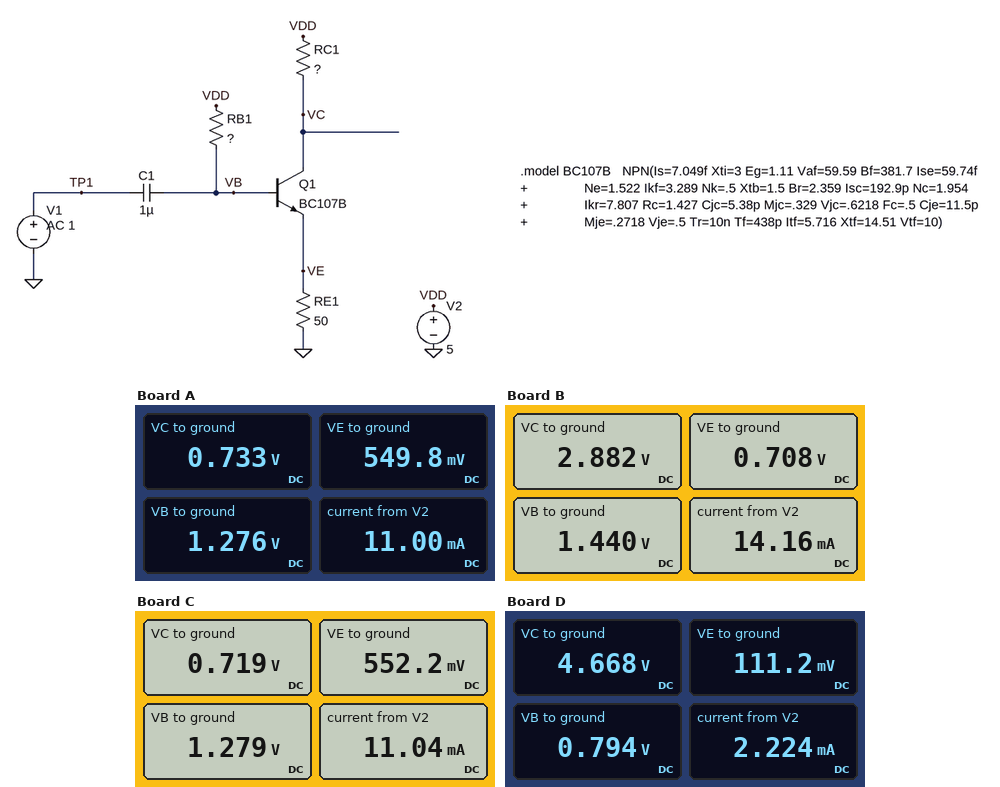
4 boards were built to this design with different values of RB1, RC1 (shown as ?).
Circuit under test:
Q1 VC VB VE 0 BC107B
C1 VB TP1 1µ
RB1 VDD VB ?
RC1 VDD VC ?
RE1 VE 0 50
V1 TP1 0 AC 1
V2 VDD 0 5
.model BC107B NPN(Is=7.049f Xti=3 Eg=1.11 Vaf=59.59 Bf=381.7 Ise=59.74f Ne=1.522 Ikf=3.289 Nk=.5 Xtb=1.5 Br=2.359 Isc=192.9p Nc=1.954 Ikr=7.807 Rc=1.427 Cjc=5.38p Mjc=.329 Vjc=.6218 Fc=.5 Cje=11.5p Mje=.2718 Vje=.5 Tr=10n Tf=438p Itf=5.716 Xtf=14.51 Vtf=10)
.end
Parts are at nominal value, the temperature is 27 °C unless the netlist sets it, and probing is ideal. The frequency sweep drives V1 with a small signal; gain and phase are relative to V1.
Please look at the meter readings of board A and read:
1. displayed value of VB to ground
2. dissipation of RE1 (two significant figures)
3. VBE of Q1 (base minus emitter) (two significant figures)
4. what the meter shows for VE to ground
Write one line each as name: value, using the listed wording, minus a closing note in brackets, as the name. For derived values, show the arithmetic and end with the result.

displayed value of VB to ground: 1.276 V
dissipation of RE1: (549.8 mV)^2 / 50 Ω = 6.0 mW
VBE of Q1 (base minus emitter): 1.276 V - 549.8 mV = 730 mV
what the meter shows for VE to ground: 549.8 mV
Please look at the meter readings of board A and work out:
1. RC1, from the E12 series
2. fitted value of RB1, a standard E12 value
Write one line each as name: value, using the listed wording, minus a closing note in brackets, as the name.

RC1, from the E12 series: 390 Ω
fitted value of RB1, a standard E12 value: 68 kΩ
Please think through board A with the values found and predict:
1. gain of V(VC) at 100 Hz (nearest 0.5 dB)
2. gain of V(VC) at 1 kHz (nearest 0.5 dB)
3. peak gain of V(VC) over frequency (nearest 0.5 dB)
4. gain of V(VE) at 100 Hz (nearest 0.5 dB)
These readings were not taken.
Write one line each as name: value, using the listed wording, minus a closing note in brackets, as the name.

gain of V(VC) at 100 Hz: 0 dB
gain of V(VC) at 1 kHz: 14.0 dB
peak gain of V(VC) over frequency: 15.5 dB
gain of V(VE) at 100 Hz: -16.0 dB
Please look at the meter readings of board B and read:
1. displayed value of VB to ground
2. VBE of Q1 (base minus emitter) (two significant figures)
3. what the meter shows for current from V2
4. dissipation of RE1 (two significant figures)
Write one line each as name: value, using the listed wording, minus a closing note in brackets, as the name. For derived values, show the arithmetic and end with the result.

displayed value of VB to ground: 1.440 V
VBE of Q1 (base minus emitter): 1.44 V - 708 mV = 730 mV
what the meter shows for current from V2: 14.16 mA
dissipation of RE1: (708 mV)^2 / 50 Ω = 10 mW
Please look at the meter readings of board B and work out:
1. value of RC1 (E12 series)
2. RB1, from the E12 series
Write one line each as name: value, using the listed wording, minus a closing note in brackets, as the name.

value of RC1: 150 Ω
RB1, from the E12 series: 82 kΩ
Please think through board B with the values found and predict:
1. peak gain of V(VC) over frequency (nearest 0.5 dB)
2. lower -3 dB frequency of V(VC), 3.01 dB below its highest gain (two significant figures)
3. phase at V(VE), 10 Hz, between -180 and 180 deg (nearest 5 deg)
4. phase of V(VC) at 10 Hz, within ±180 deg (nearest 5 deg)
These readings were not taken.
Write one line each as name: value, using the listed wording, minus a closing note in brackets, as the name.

peak gain of V(VC) over frequency: 9.0 dB
lower -3 dB frequency of V(VC), 3.01 dB below its highest gain: 11 Hz
phase at V(VE), 10 Hz, between -180 and 180 deg: 50 deg
phase of V(VC) at 10 Hz, within ±180 deg: -130 deg
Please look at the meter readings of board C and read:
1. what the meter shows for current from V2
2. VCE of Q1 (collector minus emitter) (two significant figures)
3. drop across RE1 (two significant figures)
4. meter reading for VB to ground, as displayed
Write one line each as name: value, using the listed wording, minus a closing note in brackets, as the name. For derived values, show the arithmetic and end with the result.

what the meter shows for current from V2: 11.04 mA
VCE of Q1 (collector minus emitter): 719 mV - 552.2 mV = 170 mV
drop across RE1: 552.2 mV = 550 mV
meter reading for VB to ground, as displayed: 1.279 V
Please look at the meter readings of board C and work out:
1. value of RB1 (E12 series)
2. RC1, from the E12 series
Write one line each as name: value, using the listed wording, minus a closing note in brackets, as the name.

value of RB1: 56 kΩ
RC1, from the E12 series: 390 Ω
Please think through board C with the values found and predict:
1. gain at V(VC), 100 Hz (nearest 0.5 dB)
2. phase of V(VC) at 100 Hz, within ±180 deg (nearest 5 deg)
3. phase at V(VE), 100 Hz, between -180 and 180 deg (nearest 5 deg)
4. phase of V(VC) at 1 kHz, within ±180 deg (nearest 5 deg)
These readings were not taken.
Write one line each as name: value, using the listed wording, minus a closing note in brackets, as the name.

gain at V(VC), 100 Hz: -4.5 dB
phase of V(VC) at 100 Hz, within ±180 deg: -95 deg
phase at V(VE), 100 Hz, between -180 and 180 deg: 85 deg
phase of V(VC) at 1 kHz, within ±180 deg: -140 deg
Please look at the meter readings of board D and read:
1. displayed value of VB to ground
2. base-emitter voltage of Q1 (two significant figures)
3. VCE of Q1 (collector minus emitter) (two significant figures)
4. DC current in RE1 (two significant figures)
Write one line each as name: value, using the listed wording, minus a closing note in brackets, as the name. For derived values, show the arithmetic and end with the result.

displayed value of VB to ground: 0.794 V
base-emitter voltage of Q1: 794 mV - 111.2 mV = 680 mV
VCE of Q1 (collector minus emitter): 4.668 V - 111.2 mV = 4.6 V
DC current in RE1: (111.2 mV) / 50 Ω = 2.2 mA
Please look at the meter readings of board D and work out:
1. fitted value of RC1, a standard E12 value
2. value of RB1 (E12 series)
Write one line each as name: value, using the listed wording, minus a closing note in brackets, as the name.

fitted value of RC1, a standard E12 value: 150 Ω
value of RB1: 560 kΩ
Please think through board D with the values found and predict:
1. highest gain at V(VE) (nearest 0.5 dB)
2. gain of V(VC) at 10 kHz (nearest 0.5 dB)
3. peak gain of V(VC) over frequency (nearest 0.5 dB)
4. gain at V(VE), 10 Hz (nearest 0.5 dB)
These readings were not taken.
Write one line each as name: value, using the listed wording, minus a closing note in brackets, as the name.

highest gain at V(VE): -2.0 dB
gain of V(VC) at 10 kHz: 7.5 dB
peak gain of V(VC) over frequency: 7.5 dB
gain at V(VE), 10 Hz: -4.0 dB
